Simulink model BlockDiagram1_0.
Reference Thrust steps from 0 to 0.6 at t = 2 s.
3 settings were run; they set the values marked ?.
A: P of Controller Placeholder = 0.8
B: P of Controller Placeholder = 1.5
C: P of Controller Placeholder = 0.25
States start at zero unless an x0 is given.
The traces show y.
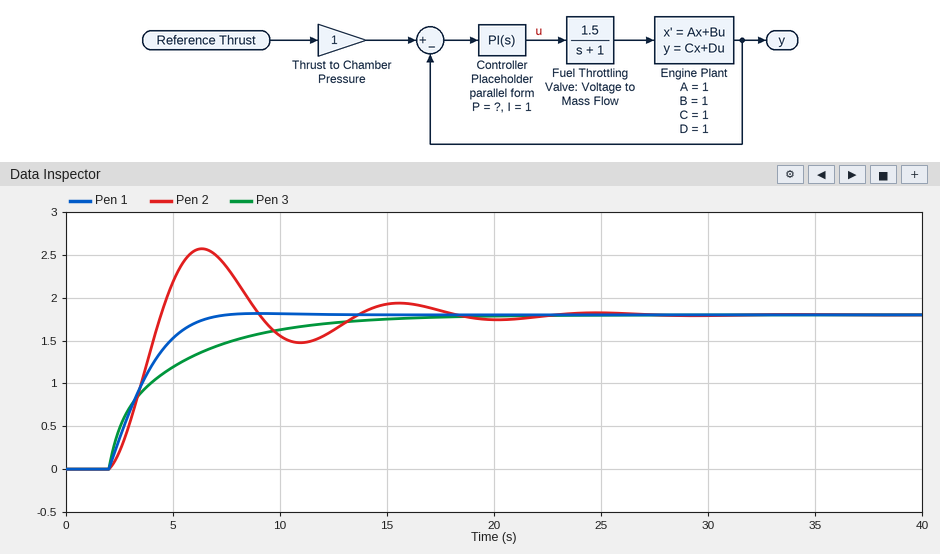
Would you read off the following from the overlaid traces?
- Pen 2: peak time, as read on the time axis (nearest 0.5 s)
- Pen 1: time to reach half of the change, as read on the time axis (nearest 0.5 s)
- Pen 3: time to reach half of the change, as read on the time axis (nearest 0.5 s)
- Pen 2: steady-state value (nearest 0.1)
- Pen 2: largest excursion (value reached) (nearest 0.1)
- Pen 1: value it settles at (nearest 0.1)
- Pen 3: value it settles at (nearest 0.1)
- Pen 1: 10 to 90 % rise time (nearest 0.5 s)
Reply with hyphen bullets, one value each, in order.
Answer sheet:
- 6.5 s
- 3.5 s
- 3.5 s
- 1.8
- 2.6
- 1.8
- 1.8
- 3.0 s
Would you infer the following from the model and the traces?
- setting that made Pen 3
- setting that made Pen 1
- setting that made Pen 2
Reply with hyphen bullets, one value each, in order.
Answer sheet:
- B
- A
- C
